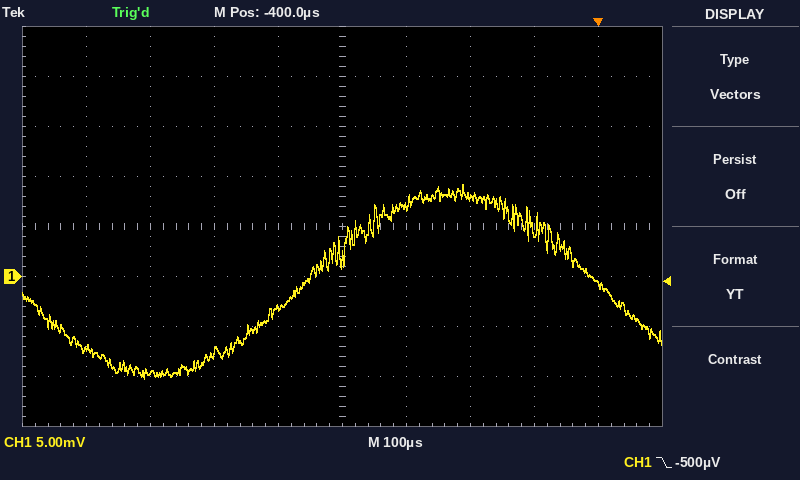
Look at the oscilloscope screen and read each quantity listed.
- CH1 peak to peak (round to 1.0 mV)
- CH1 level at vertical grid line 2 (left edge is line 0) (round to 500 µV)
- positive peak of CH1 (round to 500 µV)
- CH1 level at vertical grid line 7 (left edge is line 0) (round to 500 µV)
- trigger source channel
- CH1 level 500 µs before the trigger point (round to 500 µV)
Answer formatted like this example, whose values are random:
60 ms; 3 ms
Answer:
19.0 mV; -9.5 mV; 9.0 mV; 8.0 mV; CH1; -3.0 mV
